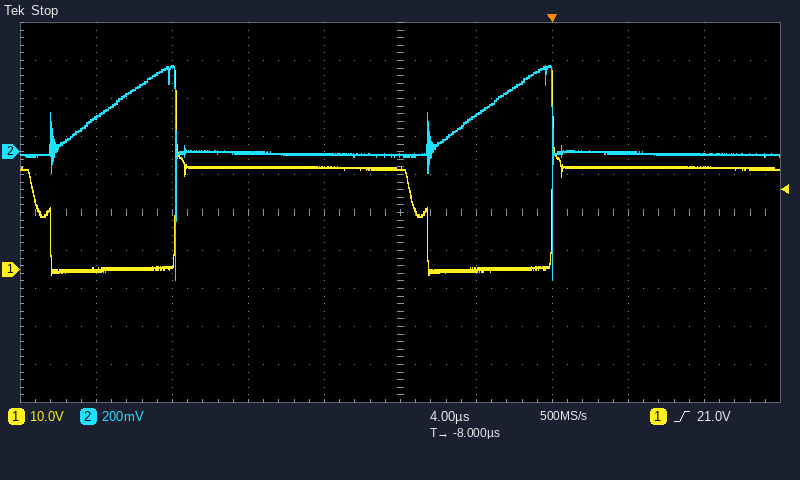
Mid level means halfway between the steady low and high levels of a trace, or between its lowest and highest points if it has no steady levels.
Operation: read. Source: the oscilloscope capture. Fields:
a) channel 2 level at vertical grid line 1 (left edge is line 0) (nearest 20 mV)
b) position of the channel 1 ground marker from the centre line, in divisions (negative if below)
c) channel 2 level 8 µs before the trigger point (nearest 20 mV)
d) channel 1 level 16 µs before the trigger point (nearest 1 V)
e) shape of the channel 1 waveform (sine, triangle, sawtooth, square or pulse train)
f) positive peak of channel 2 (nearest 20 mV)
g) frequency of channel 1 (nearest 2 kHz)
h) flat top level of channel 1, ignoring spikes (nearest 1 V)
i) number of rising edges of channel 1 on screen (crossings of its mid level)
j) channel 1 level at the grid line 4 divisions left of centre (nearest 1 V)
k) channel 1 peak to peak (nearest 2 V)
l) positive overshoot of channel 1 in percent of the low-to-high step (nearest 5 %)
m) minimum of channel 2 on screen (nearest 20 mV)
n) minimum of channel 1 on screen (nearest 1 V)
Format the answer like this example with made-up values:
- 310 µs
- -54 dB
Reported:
- 180 mV
- -1.5 div
- -20 mV
- 27 V
- pulse train
- 460 mV
- 50 kHz
- 27 V
- 2
- 0 V
- 54 V
- 95 %
- -680 mV
- -1 V
